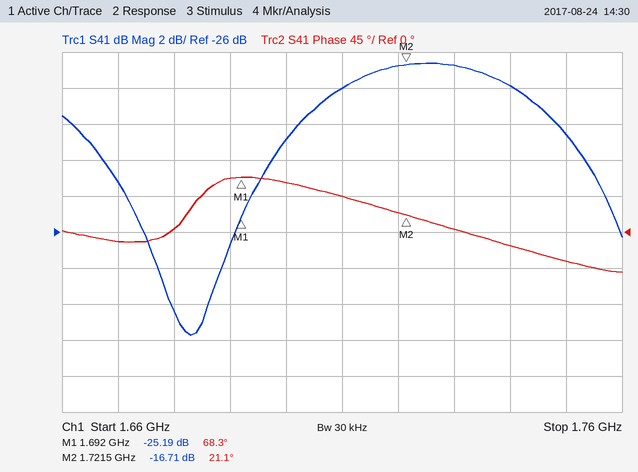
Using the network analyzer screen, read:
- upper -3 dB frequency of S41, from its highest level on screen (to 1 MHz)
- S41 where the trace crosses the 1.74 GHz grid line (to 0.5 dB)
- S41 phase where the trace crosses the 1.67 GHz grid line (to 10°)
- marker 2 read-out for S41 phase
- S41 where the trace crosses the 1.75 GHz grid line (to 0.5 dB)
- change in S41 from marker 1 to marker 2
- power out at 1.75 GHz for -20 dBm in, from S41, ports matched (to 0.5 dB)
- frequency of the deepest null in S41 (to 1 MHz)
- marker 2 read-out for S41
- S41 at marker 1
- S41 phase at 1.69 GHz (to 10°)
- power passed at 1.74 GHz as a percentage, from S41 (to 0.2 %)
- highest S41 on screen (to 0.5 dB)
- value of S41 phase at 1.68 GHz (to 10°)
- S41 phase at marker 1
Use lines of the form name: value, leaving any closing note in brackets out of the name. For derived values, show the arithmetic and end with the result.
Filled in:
upper -3 dB frequency of S41, from its highest level on screen: 1.747 GHz
S41 where the trace crosses the 1.74 GHz grid line: -18.0 dB
S41 phase where the trace crosses the 1.67 GHz grid line: -10°
marker 2 read-out for S41 phase: 21.1°
S41 where the trace crosses the 1.75 GHz grid line: -20.5 dB
change in S41 from marker 1 to marker 2: -16.71 − (-25.19) = 8.48 dB
power out at 1.75 GHz for -20 dBm in, from S41, ports matched: -20 dBm + (-20.5 dB) = -40.5 dBm
frequency of the deepest null in S41: 1.683 GHz
marker 2 read-out for S41: -16.71 dB
S41 at marker 1: -25.19 dB
S41 phase at 1.69 GHz: 70°
power passed at 1.74 GHz as a percentage, from S41: 10^(-18/10) ≈ 1.6 %
highest S41 on screen: -16.5 dB
value of S41 phase at 1.68 GHz: 0°
S41 phase at marker 1: 68.3°
